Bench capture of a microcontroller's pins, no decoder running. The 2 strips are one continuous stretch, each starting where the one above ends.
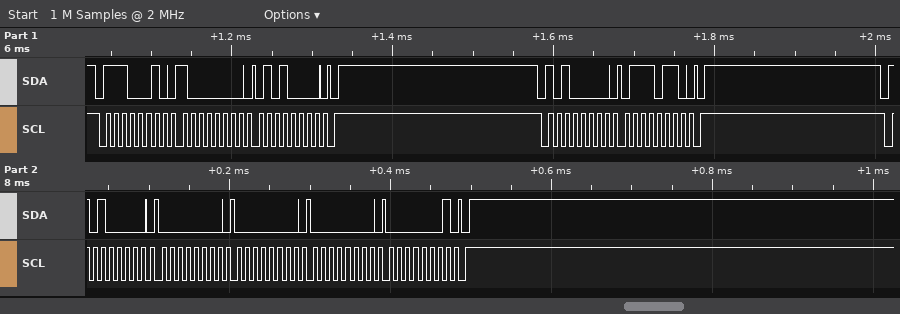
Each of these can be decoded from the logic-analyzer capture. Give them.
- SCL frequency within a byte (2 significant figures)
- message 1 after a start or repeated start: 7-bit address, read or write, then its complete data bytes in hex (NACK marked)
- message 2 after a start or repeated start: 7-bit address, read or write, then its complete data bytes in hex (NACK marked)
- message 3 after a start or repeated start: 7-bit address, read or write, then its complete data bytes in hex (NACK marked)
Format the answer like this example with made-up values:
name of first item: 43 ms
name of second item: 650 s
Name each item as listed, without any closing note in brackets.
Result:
SCL frequency within a byte: 100 kHz
message 1 after a start or repeated start: 7-bit address, read or write, then its complete data bytes in hex: 0x71 write: 80 50
message 2 after a start or repeated start: 7-bit address, read or write, then its complete data bytes in hex: 0x50 write: 76
message 3 after a start or repeated start: 7-bit address, read or write, then its complete data bytes in hex: 0x50 write: 00 00 00 01
